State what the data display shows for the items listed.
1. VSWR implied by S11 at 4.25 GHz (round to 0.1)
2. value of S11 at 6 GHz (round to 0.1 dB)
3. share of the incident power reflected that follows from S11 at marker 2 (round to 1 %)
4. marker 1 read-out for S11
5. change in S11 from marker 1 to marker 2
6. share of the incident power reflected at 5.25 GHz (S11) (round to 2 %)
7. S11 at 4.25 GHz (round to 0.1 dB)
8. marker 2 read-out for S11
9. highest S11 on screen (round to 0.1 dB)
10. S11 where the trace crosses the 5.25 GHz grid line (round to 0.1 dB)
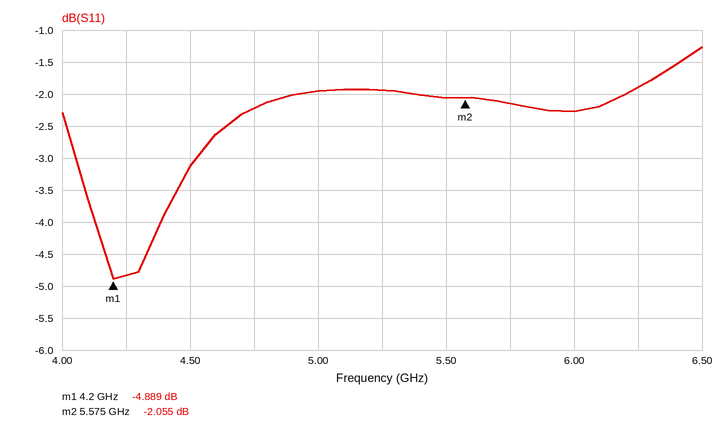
3.7
-2.3 dB
62 %
-4.889 dB
2.834 dB
64 %
-4.8 dB
-2.055 dB
-1.3 dB
-1.9 dB
